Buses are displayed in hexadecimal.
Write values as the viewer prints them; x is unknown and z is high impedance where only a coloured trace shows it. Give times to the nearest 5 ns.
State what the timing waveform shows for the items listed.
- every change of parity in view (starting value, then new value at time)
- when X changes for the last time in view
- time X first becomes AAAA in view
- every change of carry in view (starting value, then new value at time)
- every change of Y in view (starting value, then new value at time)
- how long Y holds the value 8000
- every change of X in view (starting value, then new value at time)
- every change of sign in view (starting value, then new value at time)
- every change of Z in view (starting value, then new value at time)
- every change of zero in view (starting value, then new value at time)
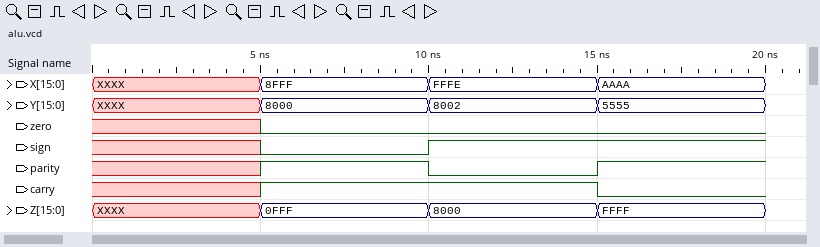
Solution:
x, 1 at 5 ns, 0 at 10 ns, 1 at 15 ns
15 ns
15 ns
x, 1 at 5 ns, 0 at 15 ns
XXXX, 8000 at 5 ns, 8002 at 10 ns, 5555 at 15 ns
5 ns
XXXX, 8FFF at 5 ns, FFFE at 10 ns, AAAA at 15 ns
x, 0 at 5 ns, 1 at 10 ns
XXXX, 0FFF at 5 ns, 8000 at 10 ns, FFFF at 15 ns
x, 0 at 5 ns
